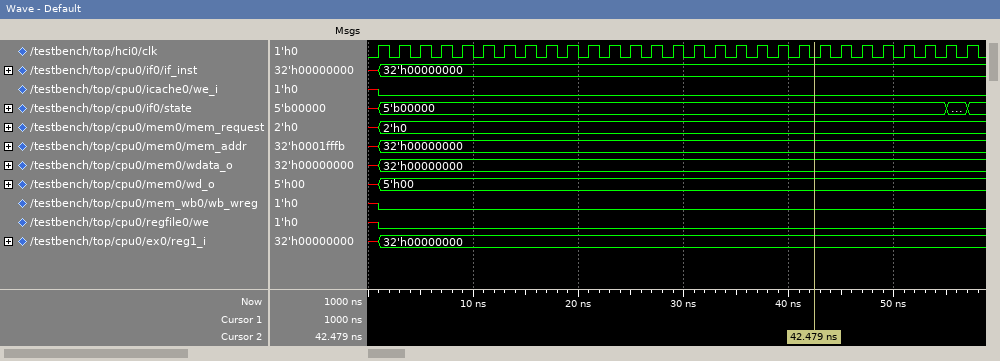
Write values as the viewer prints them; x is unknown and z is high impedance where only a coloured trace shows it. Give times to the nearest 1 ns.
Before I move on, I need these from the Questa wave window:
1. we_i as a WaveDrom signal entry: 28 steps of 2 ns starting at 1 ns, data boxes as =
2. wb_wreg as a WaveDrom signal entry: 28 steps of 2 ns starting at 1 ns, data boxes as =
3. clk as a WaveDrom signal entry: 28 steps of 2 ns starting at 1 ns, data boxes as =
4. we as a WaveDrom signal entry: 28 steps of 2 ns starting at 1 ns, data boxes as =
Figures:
{name: 'we_i', wave: '0...........................'}
{name: 'wb_wreg', wave: '0...........................'}
{name: 'clk', wave: 'p...........................'}
{name: 'we', wave: '0...........................'}
